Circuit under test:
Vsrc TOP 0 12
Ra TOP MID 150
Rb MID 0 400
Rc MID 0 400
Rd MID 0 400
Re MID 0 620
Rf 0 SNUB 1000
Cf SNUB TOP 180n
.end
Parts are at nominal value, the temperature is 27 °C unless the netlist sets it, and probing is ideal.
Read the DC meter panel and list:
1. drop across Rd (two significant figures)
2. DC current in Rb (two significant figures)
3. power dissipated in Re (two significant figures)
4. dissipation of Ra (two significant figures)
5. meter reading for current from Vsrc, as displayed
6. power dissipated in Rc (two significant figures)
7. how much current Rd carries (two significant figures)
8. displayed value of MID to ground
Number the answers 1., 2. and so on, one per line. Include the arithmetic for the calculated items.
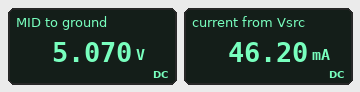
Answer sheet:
1. 5.07 V = 5.1 V
2. (5.07 V) / 400 Ω = 13 mA
3. (5.07 V)^2 / 620 Ω = 41 mW
4. (12 V - 5.07 V)^2 / 150 Ω = 320 mW
5. 46.20 mA
6. (5.07 V)^2 / 400 Ω = 64 mW
7. (5.07 V) / 400 Ω = 13 mA
8. 5.070 V
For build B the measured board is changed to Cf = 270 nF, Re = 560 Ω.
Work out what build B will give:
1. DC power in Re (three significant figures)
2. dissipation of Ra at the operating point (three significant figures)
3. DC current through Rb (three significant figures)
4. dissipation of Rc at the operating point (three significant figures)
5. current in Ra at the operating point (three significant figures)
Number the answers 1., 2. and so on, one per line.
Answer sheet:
1. 44.9 mW
2. 325 mW
3. 12.5 mA
4. 62.9 mW
5. 46.6 mA
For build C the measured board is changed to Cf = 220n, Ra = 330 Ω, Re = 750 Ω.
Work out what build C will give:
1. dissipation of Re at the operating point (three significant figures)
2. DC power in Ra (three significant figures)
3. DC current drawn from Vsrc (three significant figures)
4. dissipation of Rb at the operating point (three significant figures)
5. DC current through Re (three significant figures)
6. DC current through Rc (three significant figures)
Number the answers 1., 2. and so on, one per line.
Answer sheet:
1. 12.5 mW
2. 242 mW
3. 27.1 mA
4. 23.5 mW
5. 4.09 mA
6. 7.66 mA
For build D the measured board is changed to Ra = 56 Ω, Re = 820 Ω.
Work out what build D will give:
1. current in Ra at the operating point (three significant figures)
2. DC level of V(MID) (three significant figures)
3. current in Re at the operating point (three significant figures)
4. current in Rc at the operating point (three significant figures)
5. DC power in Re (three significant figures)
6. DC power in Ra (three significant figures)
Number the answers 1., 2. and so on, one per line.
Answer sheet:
1. 70.3 mA
2. 8.06 V
3. 9.83 mA
4. 20.2 mA
5. 79.3 mW
6. 277 mW
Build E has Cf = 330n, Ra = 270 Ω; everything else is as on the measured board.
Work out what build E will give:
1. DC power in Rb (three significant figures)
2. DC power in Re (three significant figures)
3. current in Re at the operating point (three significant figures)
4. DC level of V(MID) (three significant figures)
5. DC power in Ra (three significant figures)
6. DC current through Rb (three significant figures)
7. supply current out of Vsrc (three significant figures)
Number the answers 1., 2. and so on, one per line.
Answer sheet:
1. 30.1 mW
2. 19.4 mW
3. 5.59 mA
4. 3.47 V
5. 270 mW
6. 8.67 mA
7. 31.6 mA
